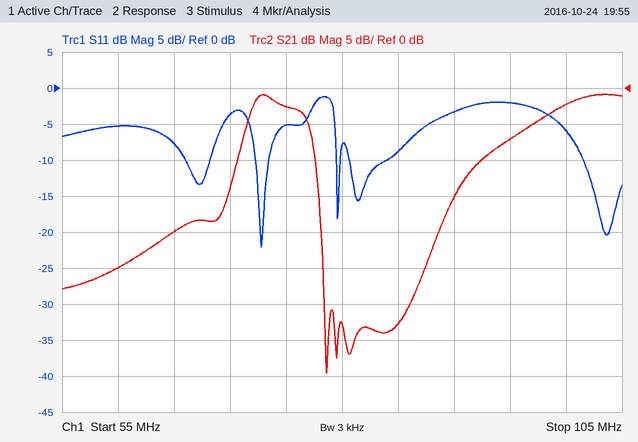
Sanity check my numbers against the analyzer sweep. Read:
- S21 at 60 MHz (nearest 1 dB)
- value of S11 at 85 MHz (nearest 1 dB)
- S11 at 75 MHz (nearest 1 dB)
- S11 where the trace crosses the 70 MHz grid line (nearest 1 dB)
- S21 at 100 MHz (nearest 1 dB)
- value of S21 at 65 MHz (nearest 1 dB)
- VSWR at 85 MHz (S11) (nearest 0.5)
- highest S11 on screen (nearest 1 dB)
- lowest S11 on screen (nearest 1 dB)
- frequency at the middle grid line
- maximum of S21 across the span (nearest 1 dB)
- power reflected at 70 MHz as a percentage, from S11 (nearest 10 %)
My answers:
-25 dB
-9 dB
-5 dB
-4 dB
-2 dB
-20 dB
2.0
-1 dB
-22 dB
80 MHz
-1 dB
40 %
